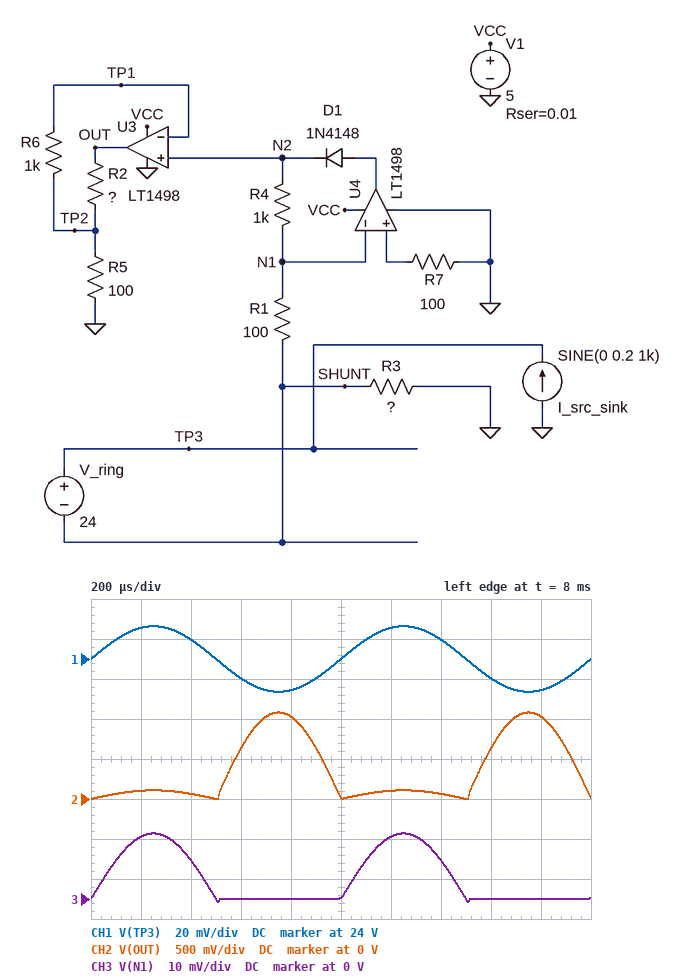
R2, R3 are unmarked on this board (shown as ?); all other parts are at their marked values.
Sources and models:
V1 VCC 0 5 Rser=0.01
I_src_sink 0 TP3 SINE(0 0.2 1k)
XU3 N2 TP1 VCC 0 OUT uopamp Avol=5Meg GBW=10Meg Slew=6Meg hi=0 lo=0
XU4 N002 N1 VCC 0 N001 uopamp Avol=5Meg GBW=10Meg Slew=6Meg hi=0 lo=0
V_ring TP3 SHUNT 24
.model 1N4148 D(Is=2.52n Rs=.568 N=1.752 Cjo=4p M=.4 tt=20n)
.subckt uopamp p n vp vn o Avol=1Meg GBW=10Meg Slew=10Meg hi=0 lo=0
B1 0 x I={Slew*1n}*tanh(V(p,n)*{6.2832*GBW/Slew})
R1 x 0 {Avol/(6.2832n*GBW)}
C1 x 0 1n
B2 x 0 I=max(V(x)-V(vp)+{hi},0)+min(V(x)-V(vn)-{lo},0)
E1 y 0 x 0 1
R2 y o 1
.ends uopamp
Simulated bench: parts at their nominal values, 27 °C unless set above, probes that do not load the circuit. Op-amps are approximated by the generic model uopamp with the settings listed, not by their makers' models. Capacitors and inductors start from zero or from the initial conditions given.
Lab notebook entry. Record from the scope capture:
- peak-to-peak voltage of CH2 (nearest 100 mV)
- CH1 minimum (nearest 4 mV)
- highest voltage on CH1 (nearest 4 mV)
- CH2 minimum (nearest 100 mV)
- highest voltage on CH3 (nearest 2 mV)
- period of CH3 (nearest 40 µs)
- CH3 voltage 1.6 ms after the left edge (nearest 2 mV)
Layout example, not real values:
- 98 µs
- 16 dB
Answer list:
- 1.1 V
- 23.984 V
- 24.016 V
- 0 V
- 16 mV
- 1.00 ms
- 0 V
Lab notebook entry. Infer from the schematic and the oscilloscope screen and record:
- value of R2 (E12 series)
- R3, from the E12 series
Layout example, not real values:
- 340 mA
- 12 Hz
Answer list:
- 560 Ω
- 0.082 Ω
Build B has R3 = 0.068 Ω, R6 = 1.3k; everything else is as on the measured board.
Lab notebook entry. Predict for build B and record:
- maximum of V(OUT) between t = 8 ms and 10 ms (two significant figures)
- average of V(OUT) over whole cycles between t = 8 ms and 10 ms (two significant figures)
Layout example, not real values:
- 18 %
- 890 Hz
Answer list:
- 900 mV
- 310 mV
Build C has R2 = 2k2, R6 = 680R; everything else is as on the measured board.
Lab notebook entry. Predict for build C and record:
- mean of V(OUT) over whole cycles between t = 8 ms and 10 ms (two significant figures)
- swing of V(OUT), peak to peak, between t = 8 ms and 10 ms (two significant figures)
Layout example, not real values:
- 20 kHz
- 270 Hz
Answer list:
- 1.3 V
- 3.8 V
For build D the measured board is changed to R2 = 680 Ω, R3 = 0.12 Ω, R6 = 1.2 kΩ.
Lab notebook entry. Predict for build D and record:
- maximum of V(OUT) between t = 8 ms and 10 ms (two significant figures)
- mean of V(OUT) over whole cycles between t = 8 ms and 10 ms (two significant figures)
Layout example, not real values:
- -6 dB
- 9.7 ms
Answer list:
- 1.9 V
- 650 mV
